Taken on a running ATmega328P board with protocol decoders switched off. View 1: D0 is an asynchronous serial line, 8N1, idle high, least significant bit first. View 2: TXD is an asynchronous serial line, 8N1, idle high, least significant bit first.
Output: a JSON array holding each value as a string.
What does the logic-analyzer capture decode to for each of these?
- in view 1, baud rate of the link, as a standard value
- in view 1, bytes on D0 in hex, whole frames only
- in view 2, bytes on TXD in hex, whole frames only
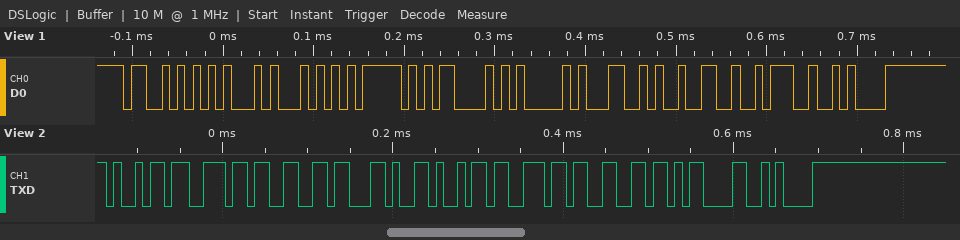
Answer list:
["115200 baud", "0x53 0x45 0x54 0x5F 0x43 0x41 0x4C 0x32 0x3A 0x0A", "69 6E 66 2C 69 6E 66 0D 0A"]
